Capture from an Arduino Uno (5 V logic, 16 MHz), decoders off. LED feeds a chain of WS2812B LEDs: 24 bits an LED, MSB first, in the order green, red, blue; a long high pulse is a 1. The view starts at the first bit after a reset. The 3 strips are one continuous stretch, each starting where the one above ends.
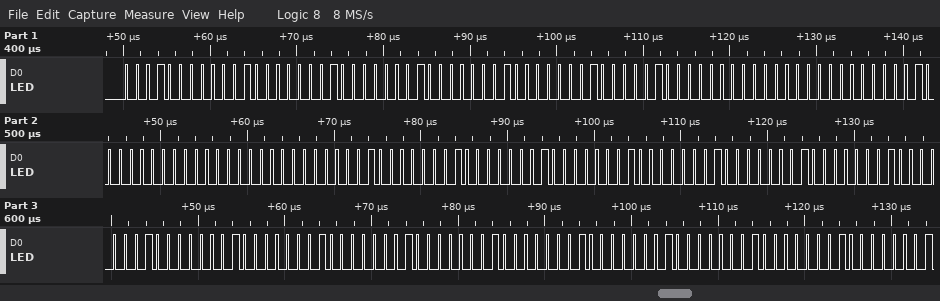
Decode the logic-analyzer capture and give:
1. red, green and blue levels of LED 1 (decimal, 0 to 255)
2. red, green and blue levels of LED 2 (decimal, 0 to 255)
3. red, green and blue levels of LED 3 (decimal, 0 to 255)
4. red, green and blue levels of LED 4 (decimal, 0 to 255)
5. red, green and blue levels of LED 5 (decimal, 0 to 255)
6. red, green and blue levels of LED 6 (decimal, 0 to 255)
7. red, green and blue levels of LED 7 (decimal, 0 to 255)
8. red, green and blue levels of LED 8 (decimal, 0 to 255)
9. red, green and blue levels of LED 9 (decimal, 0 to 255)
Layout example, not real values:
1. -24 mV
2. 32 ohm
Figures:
1. 16, 16, 16
2. 16, 16, 16
3. 0, 64, 0
4. 0, 64, 0
5. 16, 16, 16
6. 16, 16, 16
7. 16, 16, 16
8. 16, 16, 16
9. 16, 16, 16
